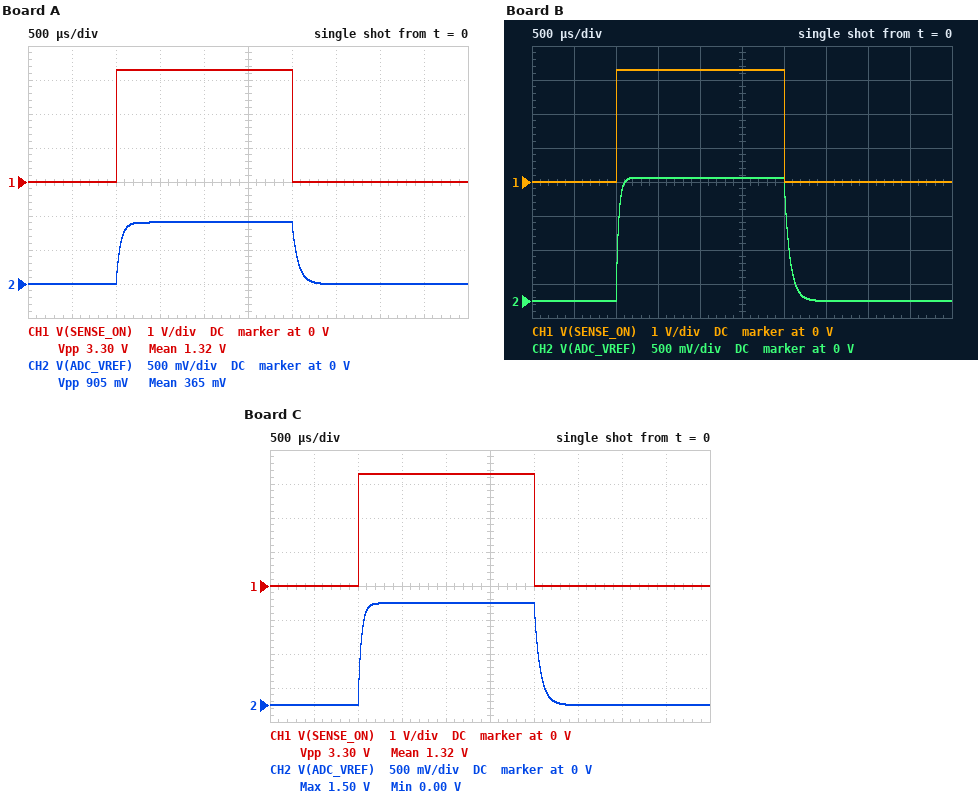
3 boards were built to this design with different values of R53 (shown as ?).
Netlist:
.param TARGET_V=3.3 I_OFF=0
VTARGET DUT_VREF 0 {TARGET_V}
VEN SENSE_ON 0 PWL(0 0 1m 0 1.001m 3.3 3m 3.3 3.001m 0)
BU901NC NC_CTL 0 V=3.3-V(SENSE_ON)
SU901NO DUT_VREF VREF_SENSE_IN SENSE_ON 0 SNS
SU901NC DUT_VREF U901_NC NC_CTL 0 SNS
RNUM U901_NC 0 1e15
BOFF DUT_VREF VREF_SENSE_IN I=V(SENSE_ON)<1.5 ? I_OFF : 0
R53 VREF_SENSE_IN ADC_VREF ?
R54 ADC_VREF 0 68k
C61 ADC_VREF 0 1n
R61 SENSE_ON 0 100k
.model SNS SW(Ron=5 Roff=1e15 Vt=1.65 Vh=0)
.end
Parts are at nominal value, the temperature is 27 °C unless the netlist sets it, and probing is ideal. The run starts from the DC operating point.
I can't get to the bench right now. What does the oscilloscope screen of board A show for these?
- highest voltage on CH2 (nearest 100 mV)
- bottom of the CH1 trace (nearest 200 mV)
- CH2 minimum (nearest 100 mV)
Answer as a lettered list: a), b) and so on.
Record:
a) 900 mV
b) 0 V
c) 0 V
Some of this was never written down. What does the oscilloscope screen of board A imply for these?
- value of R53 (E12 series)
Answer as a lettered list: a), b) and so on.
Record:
a) 180 kΩ
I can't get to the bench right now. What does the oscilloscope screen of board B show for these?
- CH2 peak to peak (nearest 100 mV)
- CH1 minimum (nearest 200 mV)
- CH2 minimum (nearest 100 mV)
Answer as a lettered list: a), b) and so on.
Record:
a) 1.8 V
b) 0 V
c) 0 V
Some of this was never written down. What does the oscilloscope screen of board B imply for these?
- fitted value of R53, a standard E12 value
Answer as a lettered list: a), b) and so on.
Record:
a) 56 kΩ
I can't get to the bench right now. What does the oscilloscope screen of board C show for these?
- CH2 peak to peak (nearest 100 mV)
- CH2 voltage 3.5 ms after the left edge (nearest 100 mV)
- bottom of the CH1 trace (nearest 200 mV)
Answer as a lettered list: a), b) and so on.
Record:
a) 1.5 V
b) 0 V
c) 0 V
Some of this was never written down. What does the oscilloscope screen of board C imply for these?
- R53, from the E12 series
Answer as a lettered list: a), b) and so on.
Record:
a) 82 kΩ
